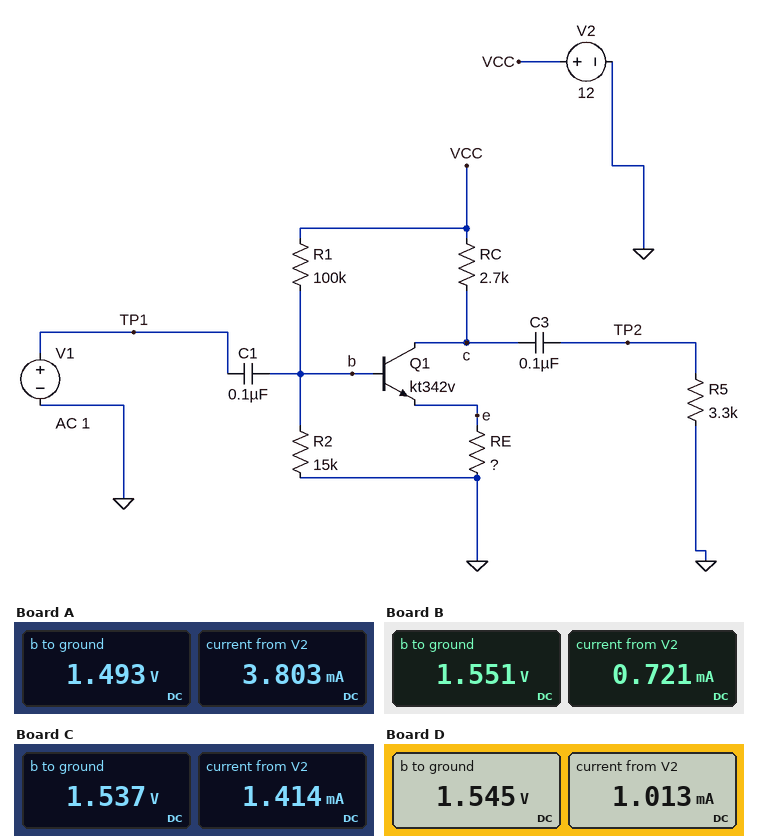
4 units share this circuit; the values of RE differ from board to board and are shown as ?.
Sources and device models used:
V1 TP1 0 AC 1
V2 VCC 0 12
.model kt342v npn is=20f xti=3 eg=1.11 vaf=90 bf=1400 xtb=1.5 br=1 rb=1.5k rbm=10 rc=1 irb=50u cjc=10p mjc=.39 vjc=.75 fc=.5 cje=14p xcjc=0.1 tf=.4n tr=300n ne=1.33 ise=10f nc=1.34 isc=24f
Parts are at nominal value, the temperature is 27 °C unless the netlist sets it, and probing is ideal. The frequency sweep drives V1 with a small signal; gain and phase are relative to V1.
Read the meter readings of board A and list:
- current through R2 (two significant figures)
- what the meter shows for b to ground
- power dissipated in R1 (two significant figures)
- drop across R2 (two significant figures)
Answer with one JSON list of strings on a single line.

["100 µA", "1.493 V", "1.1 mW", "1.5 V"]
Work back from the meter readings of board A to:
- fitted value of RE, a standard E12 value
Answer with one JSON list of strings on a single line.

["220 Ω"]
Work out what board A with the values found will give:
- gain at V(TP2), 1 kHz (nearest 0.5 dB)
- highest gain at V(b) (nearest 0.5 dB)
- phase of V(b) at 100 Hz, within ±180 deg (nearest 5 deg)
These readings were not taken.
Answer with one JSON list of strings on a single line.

["16.0 dB", "0 dB", "55 deg"]
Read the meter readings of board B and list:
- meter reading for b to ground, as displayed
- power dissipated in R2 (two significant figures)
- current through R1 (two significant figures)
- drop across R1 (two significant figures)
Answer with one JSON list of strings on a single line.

["1.551 V", "160 µW", "100 µA", "10 V"]
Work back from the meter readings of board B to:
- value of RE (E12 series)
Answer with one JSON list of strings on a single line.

["1.5 kΩ"]
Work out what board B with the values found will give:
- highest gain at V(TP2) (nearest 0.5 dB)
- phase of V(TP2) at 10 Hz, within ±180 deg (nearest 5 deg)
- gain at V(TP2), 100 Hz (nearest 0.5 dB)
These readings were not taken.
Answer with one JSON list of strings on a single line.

["-0.5 dB", "-5 deg", "-13.5 dB"]
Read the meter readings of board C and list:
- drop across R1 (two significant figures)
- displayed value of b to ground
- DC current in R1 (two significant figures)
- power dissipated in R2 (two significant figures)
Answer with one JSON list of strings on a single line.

["10 V", "1.537 V", "100 µA", "160 µW"]
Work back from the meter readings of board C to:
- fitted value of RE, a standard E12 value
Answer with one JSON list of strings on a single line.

["680 Ω"]
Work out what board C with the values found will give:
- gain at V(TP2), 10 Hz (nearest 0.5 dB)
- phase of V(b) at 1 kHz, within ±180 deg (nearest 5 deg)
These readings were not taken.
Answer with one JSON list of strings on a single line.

["-44.0 dB", "5 deg"]
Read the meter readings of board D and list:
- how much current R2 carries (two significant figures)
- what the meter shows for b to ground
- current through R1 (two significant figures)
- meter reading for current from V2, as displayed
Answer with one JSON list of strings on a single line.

["100 µA", "1.545 V", "100 µA", "1.013 mA"]
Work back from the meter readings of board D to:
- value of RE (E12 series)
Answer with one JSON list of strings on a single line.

["1 kΩ"]
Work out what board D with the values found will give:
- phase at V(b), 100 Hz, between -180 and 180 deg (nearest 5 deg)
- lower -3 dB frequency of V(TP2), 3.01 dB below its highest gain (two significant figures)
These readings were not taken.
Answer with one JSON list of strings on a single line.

["50 deg", "310 Hz"]
